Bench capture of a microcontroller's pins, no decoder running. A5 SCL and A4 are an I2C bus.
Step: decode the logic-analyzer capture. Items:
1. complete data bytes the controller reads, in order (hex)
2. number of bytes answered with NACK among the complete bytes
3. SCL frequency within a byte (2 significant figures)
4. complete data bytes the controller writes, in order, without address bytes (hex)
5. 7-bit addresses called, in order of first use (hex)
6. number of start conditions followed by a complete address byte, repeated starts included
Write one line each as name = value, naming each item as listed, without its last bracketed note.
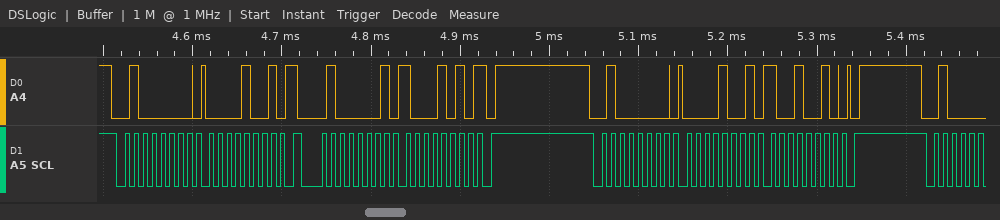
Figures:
complete data bytes the controller reads, in order = 8A
number of bytes answered with NACK among the complete bytes = 1
SCL frequency within a byte = 100 kHz
complete data bytes the controller writes, in order, without address bytes = 09 09 92
7-bit addresses called, in order of first use = 0x20
number of start conditions followed by a complete address byte, repeated starts included = 3
